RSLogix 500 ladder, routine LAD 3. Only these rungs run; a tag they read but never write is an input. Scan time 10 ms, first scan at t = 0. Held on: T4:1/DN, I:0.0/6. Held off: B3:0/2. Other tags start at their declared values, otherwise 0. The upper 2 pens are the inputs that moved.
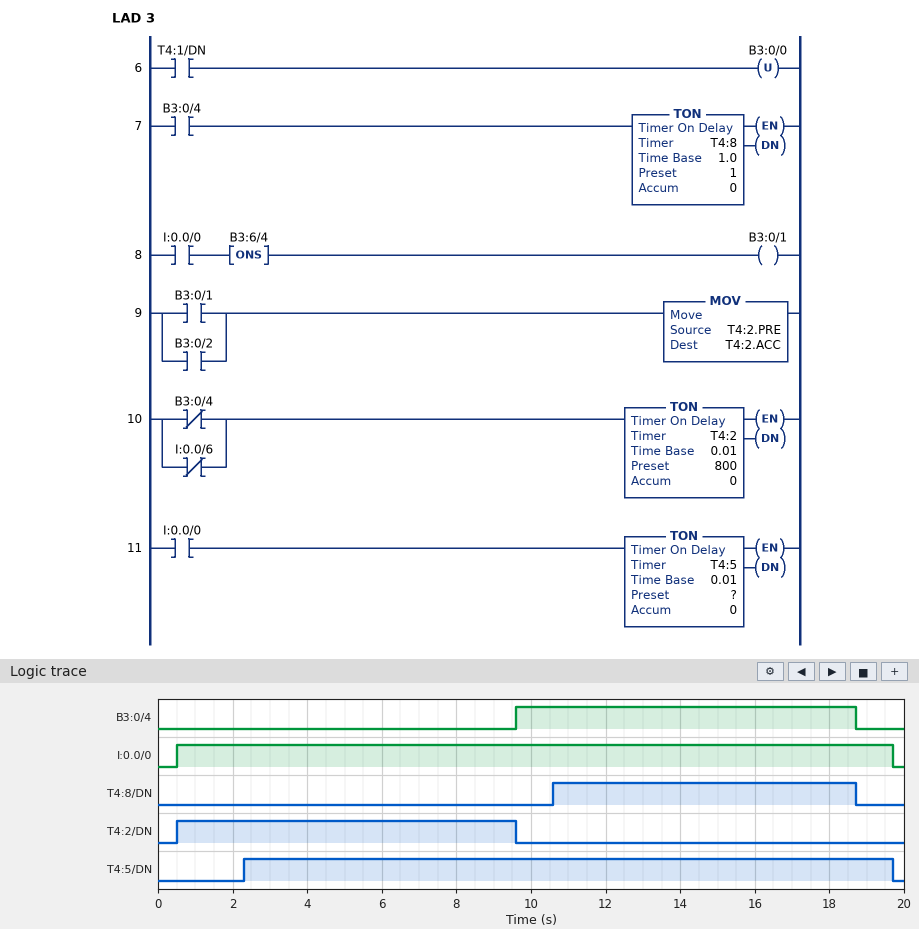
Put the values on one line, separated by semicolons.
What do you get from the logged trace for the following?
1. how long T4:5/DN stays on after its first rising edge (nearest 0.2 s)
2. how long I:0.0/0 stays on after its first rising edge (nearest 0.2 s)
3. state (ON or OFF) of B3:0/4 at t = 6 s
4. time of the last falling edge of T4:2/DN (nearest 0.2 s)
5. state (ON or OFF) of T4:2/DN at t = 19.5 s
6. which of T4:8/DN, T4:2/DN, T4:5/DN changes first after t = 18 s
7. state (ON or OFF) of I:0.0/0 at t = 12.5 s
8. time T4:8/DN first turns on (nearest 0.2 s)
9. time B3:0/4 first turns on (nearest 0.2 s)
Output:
17.4 s; 19.2 s; OFF; 9.6 s; OFF; T4:8/DN; ON; 10.6 s; 9.6 s
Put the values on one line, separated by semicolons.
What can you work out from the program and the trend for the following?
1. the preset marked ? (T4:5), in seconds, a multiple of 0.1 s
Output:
1.8 s
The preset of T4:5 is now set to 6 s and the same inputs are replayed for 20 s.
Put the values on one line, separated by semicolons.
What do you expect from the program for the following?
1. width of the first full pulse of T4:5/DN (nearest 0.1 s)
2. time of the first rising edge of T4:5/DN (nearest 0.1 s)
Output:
13.2 s; 6.5 s
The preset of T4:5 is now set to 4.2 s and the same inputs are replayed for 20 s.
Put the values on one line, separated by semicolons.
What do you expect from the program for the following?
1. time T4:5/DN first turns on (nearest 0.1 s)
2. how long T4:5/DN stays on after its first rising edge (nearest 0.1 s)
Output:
4.7 s; 15.0 s
